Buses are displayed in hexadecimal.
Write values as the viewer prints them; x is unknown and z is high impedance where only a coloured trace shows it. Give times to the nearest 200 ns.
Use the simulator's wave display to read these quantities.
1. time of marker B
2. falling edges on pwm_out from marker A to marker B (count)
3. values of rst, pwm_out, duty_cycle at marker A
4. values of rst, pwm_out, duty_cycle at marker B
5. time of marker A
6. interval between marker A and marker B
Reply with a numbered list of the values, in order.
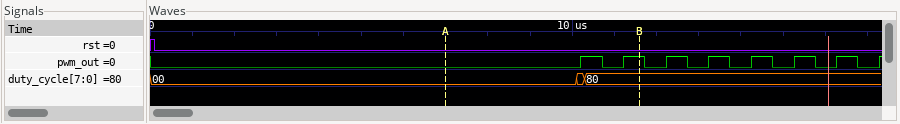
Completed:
1. 11600 ns
2. 1
3. rst=0, pwm_out=0, duty_cycle=00
4. rst=0, pwm_out=1, duty_cycle=80
5. 7000 ns
6. 4600 ns
